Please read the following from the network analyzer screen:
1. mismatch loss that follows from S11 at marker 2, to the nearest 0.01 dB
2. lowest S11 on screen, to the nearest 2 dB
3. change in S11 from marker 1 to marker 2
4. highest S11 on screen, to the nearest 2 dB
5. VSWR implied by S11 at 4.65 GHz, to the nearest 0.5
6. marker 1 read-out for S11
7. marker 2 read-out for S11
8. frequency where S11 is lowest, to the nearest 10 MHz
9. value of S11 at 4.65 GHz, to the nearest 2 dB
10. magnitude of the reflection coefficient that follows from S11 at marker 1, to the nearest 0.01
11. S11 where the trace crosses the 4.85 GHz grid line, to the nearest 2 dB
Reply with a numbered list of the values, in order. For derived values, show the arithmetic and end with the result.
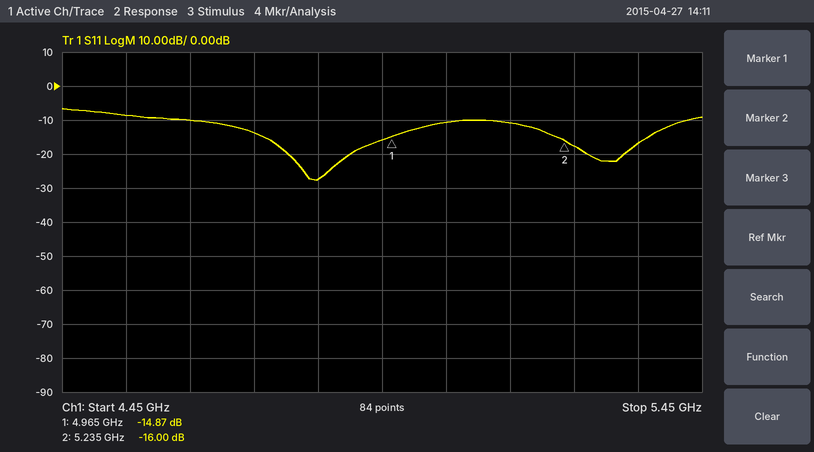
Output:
1. −10 log10(1 − 10^(-16/10)) ≈ 0.11 dB
2. -28 dB
3. -16 − (-14.87) = -1.13 dB
4. -6 dB
5. |Γ| = 10^(-10/20) = 0.3162; VSWR = (1 + 0.3162)/(1 − 0.3162) ≈ 1.92, so 2.0 to the nearest 0.5
6. -14.87 dB
7. -16.00 dB
8. 4.85 GHz
9. -10 dB
10. 10^(-14.87/20) ≈ 0.18
11. -28 dB
